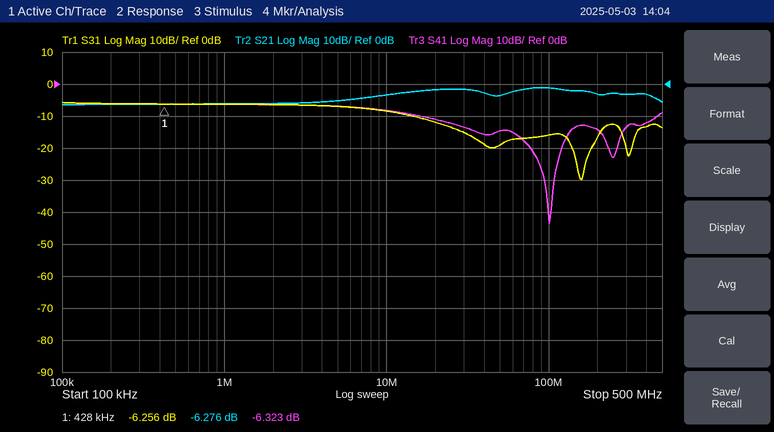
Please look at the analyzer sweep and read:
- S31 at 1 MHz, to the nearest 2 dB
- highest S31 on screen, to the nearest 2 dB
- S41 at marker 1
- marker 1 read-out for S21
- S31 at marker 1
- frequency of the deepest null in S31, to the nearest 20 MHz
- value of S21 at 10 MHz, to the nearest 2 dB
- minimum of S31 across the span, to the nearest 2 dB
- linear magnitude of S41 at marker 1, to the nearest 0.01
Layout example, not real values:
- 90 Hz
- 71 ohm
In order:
- -6 dB
- -6 dB
- -6.323 dB
- -6.276 dB
- -6.256 dB
- 160 MHz
- -4 dB
- -30 dB
- 0.48
